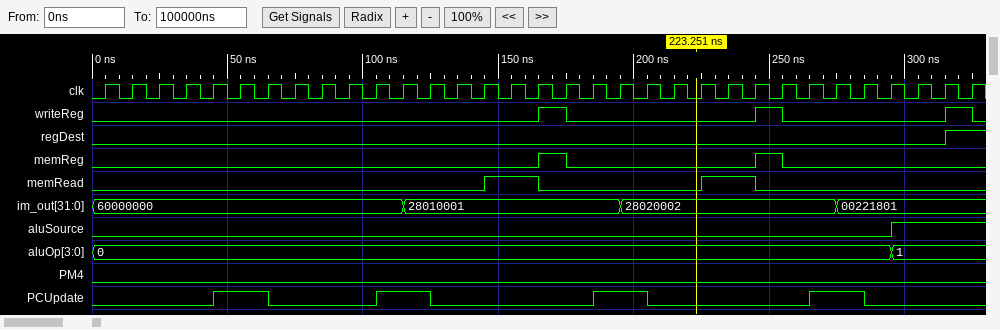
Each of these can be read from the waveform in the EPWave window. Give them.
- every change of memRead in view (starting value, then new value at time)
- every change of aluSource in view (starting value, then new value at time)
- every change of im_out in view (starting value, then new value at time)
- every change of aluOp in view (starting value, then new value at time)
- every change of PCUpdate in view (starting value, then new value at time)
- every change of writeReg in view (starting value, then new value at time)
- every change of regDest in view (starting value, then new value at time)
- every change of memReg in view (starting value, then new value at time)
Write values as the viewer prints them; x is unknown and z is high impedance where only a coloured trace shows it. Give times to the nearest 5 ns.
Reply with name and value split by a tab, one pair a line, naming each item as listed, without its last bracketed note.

every change of memRead in view	0, 1 at 145 ns, 0 at 165 ns, 1 at 225 ns, 0 at 245 ns
every change of aluSource in view	0, 1 at 295 ns
every change of im_out in view	60000000, 28010001 at 115 ns, 28020002 at 195 ns, 00221801 at 275 ns
every change of aluOp in view	0, 1 at 295 ns
every change of PCUpdate in view	0, 1 at 45 ns, 0 at 65 ns, 1 at 105 ns, 0 at 125 ns, 1 at 185 ns, 0 at 205 ns, 1 at 265 ns, 0 at 285 ns
every change of writeReg in view	0, 1 at 165 ns, 0 at 175 ns, 1 at 245 ns, 0 at 255 ns, 1 at 315 ns, 0 at 325 ns
every change of regDest in view	0, 1 at 315 ns
every change of memReg in view	0, 1 at 165 ns, 0 at 175 ns, 1 at 245 ns, 0 at 255 ns
